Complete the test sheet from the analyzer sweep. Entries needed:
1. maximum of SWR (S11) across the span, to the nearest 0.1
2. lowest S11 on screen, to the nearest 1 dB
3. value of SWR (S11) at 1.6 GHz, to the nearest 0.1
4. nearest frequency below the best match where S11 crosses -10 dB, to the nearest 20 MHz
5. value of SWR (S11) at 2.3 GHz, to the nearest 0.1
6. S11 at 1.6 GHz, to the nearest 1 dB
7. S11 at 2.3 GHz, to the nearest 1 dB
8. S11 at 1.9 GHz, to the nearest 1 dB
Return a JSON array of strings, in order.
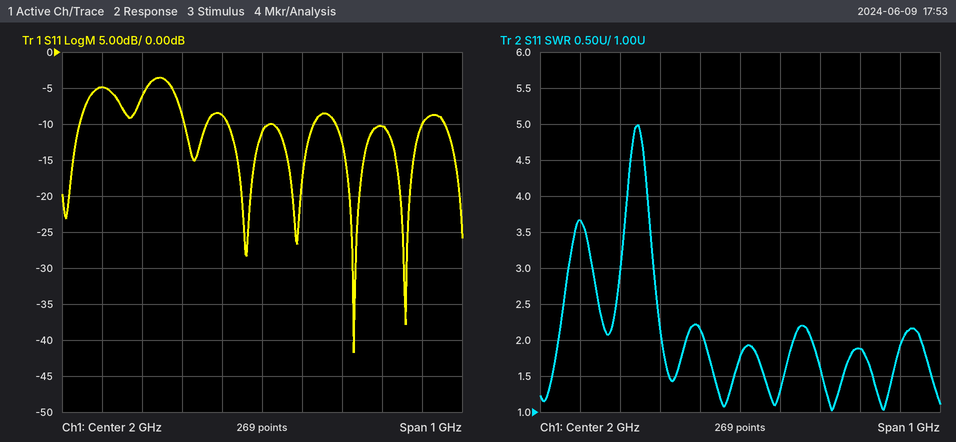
["5.0", "-42 dB", "3.7", "2.18 GHz", "1.9", "-5 dB", "-10 dB", "-9 dB"]
